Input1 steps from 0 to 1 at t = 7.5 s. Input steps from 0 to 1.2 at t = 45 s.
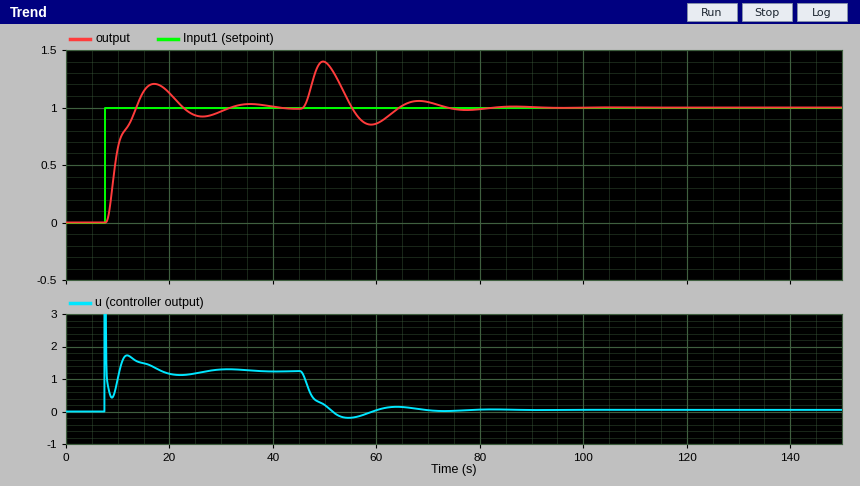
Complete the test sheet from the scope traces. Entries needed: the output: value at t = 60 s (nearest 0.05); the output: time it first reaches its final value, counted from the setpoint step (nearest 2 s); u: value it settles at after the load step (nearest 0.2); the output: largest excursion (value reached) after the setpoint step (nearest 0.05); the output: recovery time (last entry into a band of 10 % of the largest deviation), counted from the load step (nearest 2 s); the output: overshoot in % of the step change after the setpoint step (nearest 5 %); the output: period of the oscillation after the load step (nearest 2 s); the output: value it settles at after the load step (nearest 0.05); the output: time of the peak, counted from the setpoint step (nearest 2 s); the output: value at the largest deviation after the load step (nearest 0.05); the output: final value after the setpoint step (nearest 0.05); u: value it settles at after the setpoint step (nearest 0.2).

0.85
6 s
0.0
1.20
26 s
20 %
18 s
1.00
10 s
1.40
1.00
1.2
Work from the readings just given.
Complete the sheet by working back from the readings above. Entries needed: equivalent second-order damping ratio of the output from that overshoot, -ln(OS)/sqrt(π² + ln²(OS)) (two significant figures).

0.46
